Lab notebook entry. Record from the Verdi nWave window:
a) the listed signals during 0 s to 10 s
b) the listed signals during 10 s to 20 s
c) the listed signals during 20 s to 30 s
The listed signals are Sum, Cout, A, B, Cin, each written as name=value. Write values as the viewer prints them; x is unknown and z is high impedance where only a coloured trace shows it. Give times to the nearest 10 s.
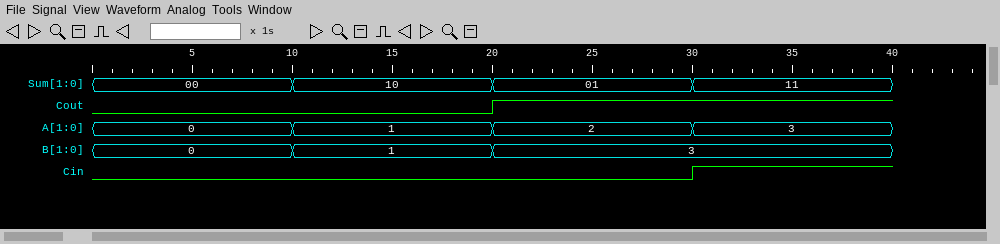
Sum=00, Cout=0, A=0, B=0, Cin=0
Sum=10, Cout=0, A=1, B=1, Cin=0
Sum=01, Cout=1, A=2, B=3, Cin=0
